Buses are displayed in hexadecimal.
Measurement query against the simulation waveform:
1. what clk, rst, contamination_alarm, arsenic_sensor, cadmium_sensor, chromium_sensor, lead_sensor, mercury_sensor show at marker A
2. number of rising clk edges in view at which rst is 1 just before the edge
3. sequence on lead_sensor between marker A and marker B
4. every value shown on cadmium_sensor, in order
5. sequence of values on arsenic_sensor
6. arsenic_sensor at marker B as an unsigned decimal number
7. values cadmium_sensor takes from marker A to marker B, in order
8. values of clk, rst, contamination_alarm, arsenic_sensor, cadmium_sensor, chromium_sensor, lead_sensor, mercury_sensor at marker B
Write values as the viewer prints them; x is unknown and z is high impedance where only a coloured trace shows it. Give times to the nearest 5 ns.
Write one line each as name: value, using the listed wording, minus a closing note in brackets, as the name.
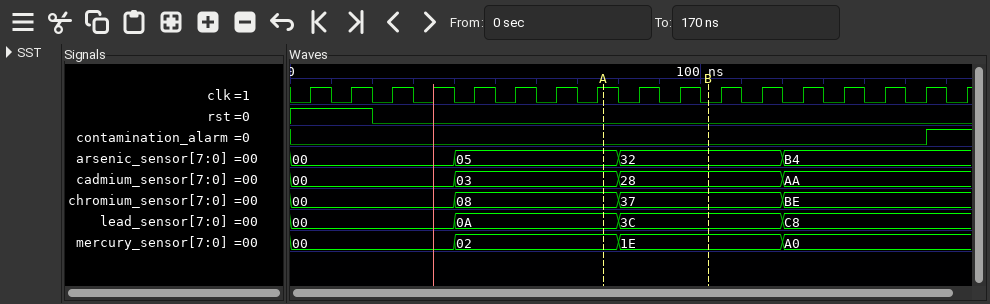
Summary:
what clk, rst, contamination_alarm, arsenic_sensor, cadmium_sensor, chromium_sensor, lead_sensor, mercury_sensor show at marker A: clk=1, rst=0, contamination_alarm=0, arsenic_sensor=05, cadmium_sensor=03, chromium_sensor=08, lead_sensor=0A, mercury_sensor=02
number of rising clk edges in view at which rst is 1 just before the edge: 2
sequence on lead_sensor between marker A and marker B: 0A, 3C
every value shown on cadmium_sensor, in order: 00, 03, 28, AA
sequence of values on arsenic_sensor: 00, 05, 32, B4
arsenic_sensor at marker B as an unsigned decimal number: 50
values cadmium_sensor takes from marker A to marker B, in order: 03, 28
values of clk, rst, contamination_alarm, arsenic_sensor, cadmium_sensor, chromium_sensor, lead_sensor, mercury_sensor at marker B: clk=0, rst=0, contamination_alarm=0, arsenic_sensor=32, cadmium_sensor=28, chromium_sensor=37, lead_sensor=3C, mercury_sensor=1E
